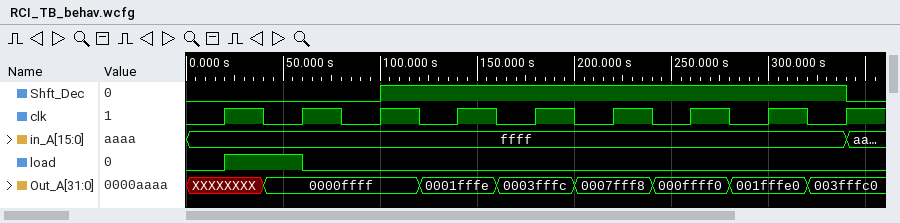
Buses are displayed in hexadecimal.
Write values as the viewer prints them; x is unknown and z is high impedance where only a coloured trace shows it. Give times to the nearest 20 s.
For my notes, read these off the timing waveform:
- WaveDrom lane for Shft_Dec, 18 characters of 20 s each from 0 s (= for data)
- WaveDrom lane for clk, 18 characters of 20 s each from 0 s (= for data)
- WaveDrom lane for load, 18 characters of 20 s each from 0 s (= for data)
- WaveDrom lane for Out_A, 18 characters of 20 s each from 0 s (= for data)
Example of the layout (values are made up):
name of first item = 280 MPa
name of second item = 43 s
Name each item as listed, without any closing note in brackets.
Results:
WaveDrom lane for Shft_Dec, 18 characters of 20 s each from 0 s = {name: 'Shft_Dec', wave: '0....1...........0'}
WaveDrom lane for clk, 18 characters of 20 s each from 0 s = {name: 'clk', wave: '010101010101010101'}
WaveDrom lane for load, 18 characters of 20 s each from 0 s = {name: 'load', wave: '01.0..............'}
WaveDrom lane for Out_A, 18 characters of 20 s each from 0 s = {name: 'Out_A', wave: 'x.=...=.=.=.=.=.=.', data: '0000ffff 0001fffe 0003fffc 0007fff8 000ffff0 001fffe0 003fffc0'}
